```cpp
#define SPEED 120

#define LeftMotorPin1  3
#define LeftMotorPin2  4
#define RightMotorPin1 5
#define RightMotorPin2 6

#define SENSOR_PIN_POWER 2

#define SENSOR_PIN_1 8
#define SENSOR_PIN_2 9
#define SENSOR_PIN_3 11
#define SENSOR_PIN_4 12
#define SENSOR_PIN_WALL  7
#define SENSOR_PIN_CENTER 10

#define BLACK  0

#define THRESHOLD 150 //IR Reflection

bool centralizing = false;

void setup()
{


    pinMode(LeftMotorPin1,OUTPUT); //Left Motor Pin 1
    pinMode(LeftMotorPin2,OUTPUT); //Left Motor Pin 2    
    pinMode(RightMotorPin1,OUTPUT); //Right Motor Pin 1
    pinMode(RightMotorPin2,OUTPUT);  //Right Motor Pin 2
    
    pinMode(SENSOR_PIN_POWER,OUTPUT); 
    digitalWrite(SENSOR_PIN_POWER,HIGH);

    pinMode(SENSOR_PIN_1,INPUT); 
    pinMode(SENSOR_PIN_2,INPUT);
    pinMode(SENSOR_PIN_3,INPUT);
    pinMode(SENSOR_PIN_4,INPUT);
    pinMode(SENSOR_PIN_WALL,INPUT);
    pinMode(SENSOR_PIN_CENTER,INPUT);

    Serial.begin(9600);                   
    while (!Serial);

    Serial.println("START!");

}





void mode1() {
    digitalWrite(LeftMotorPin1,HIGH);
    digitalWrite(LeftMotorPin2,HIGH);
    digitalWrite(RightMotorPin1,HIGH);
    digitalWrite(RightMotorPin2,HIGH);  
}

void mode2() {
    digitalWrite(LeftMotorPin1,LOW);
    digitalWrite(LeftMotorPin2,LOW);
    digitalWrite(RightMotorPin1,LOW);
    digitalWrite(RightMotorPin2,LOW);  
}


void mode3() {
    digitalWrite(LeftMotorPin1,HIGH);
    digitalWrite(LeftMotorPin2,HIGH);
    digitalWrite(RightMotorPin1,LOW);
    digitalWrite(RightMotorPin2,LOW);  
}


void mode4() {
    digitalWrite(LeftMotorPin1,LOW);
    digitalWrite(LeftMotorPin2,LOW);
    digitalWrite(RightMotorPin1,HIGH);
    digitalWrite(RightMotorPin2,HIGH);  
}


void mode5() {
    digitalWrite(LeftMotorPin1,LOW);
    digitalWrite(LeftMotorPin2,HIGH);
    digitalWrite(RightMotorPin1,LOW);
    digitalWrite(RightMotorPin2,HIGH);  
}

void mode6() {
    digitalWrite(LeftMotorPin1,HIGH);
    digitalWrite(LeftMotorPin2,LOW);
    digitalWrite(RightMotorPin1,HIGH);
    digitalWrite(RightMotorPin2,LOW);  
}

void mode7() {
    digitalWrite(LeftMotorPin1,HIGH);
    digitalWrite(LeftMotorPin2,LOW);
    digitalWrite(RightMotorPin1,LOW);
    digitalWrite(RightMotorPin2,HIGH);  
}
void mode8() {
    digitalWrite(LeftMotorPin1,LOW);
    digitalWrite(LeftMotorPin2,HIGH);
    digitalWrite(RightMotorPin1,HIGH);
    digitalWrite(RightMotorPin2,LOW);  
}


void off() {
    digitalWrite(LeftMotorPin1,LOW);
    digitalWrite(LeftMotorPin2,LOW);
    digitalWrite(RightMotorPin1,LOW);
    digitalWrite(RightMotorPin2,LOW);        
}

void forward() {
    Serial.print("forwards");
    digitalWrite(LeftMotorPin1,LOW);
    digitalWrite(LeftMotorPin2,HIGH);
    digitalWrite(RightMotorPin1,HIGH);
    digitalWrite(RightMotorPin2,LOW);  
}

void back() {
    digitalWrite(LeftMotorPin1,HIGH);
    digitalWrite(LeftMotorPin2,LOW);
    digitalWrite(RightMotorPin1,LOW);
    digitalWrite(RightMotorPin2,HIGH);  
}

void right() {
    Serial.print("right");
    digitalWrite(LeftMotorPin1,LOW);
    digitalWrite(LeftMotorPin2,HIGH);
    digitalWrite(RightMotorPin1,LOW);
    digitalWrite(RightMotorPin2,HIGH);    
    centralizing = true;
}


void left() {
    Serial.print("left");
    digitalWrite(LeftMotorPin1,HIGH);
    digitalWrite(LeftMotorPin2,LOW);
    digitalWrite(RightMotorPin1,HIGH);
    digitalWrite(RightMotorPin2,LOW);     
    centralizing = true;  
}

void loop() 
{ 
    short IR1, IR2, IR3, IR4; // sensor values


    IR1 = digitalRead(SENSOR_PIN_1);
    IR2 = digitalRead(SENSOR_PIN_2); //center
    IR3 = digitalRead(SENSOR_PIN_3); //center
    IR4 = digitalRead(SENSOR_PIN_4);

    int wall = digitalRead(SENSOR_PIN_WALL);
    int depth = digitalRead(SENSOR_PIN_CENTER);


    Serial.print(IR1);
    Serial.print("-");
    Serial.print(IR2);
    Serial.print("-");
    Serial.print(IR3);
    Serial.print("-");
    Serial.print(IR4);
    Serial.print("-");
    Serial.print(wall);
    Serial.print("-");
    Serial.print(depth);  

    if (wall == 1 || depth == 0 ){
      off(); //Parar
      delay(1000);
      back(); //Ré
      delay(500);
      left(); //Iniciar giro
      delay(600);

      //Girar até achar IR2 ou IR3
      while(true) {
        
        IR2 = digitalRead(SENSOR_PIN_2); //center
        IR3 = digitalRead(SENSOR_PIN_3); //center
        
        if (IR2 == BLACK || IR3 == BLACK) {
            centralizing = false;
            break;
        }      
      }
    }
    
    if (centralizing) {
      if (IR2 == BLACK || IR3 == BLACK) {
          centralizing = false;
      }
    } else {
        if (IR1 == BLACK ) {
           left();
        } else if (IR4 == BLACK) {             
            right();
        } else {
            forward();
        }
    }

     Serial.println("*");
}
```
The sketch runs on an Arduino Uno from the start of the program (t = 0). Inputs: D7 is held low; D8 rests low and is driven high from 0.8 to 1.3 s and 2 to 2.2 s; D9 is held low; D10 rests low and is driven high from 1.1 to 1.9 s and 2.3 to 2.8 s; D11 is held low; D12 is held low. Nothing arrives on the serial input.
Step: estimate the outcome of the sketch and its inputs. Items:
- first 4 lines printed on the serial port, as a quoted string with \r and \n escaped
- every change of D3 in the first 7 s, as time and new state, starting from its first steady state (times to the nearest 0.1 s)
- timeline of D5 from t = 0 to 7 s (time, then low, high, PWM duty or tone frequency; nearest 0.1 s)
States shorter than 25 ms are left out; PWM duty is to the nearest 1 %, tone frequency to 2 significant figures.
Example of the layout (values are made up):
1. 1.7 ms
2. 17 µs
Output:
1. "START!\r\n0-0-0-0-0-0leftleft*\r\n1-0-0-0-0-0leftright*\r\n0-0-0-0-0-0leftleft*\r\n"
2. 0 s low; 1 s high; 2.1 s low; 3.1 s high; 4.2 s low; 5.2 s high; 6.3 s low
3. 0 s low; 1.5 s high; 2.1 s low; 3.6 s high; 4.2 s low; 5.7 s high; 6.3 s low
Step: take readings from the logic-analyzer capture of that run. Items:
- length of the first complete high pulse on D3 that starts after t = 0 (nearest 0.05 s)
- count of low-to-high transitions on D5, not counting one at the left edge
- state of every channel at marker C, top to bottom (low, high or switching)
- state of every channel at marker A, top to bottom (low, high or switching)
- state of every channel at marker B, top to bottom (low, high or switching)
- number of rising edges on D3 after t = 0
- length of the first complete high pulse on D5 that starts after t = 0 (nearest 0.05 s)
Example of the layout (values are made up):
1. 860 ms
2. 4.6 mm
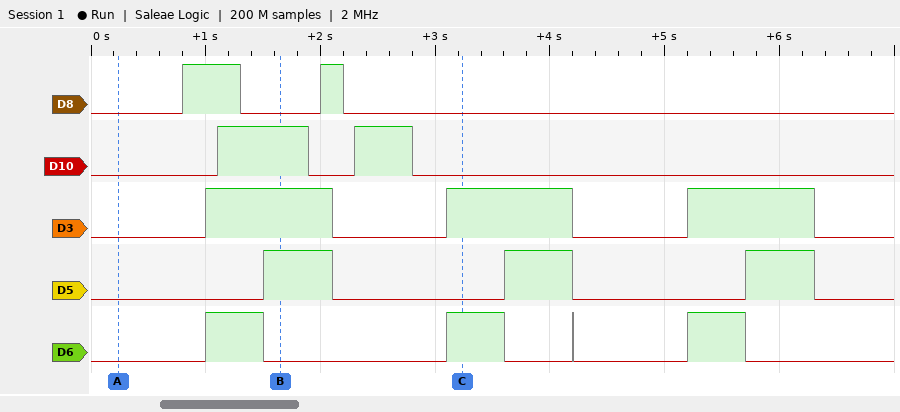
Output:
1. 1.10 s
2. 3
3. D8 low, D10 low, D3 high, D5 low, D6 high
4. D8 low, D10 low, D3 low, D5 low, D6 low
5. D8 low, D10 high, D3 high, D5 high, D6 low
6. 3
7. 0.60 s
